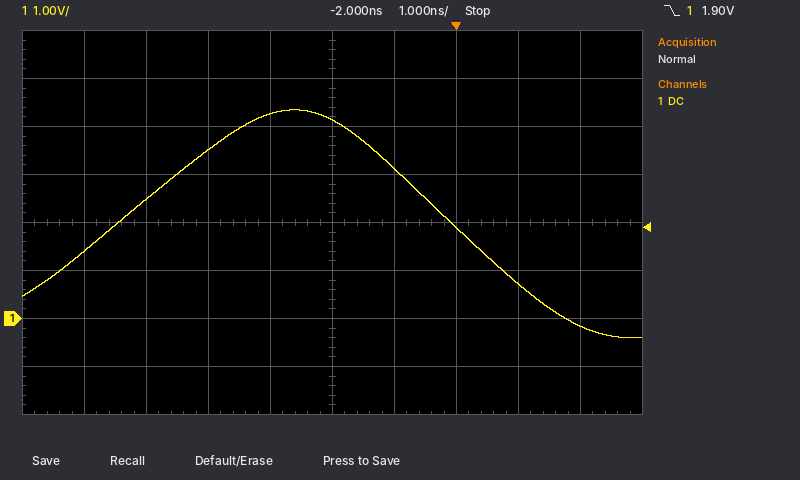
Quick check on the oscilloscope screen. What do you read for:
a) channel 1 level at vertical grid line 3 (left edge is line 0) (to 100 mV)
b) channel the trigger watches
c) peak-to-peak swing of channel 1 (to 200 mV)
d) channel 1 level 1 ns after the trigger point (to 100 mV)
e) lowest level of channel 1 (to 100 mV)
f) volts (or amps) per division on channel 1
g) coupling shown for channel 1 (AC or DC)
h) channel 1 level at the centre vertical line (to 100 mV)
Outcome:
3.5 V
channel 1
4.8 V
700 mV
-400 mV
1 V
DC
4.1 V
